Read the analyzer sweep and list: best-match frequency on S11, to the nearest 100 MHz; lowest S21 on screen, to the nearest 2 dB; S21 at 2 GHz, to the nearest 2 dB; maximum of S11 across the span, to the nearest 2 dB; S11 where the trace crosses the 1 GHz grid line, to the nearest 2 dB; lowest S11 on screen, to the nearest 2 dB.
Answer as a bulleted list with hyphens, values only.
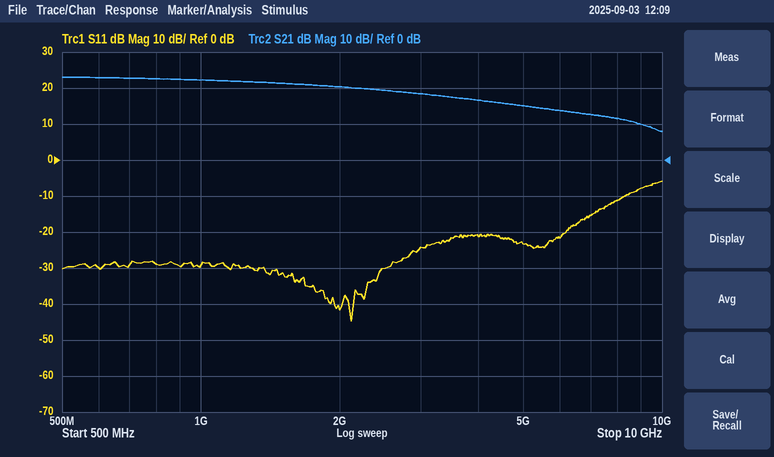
- 2.1 GHz
- 8 dB
- 20 dB
- -6 dB
- -30 dB
- -44 dB
